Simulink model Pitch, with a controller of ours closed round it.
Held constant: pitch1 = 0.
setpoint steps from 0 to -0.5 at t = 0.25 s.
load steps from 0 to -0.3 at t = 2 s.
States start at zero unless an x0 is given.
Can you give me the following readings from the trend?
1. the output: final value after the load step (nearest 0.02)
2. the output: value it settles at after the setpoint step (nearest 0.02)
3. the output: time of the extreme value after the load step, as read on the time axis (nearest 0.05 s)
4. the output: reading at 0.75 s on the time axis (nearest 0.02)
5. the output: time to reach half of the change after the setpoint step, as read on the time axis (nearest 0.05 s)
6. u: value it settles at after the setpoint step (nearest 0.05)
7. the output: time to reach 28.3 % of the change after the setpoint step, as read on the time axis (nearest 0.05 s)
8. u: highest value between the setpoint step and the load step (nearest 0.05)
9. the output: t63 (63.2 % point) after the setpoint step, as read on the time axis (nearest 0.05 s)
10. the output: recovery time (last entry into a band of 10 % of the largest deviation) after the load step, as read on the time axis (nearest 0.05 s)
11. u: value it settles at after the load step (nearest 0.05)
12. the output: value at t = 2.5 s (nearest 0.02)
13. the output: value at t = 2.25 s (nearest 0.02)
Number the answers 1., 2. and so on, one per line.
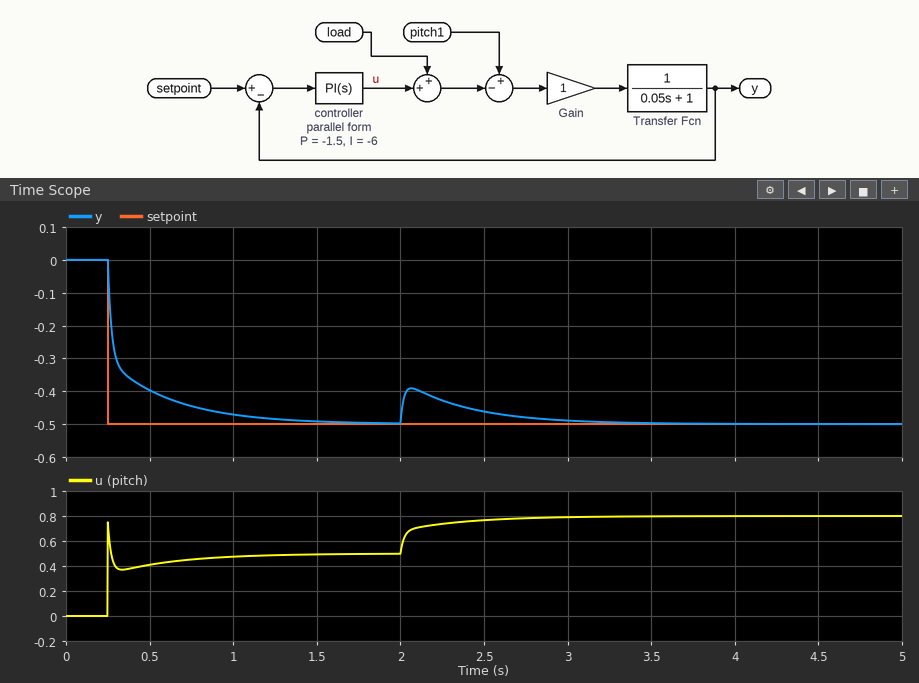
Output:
1. -0.50
2. -0.50
3. 2.05 s
4. -0.44
5. 0.30 s
6. 0.50
7. 0.25 s
8. 0.75
9. 0.30 s
10. 3.00 s
11. 0.80
12. -0.46
13. -0.42
